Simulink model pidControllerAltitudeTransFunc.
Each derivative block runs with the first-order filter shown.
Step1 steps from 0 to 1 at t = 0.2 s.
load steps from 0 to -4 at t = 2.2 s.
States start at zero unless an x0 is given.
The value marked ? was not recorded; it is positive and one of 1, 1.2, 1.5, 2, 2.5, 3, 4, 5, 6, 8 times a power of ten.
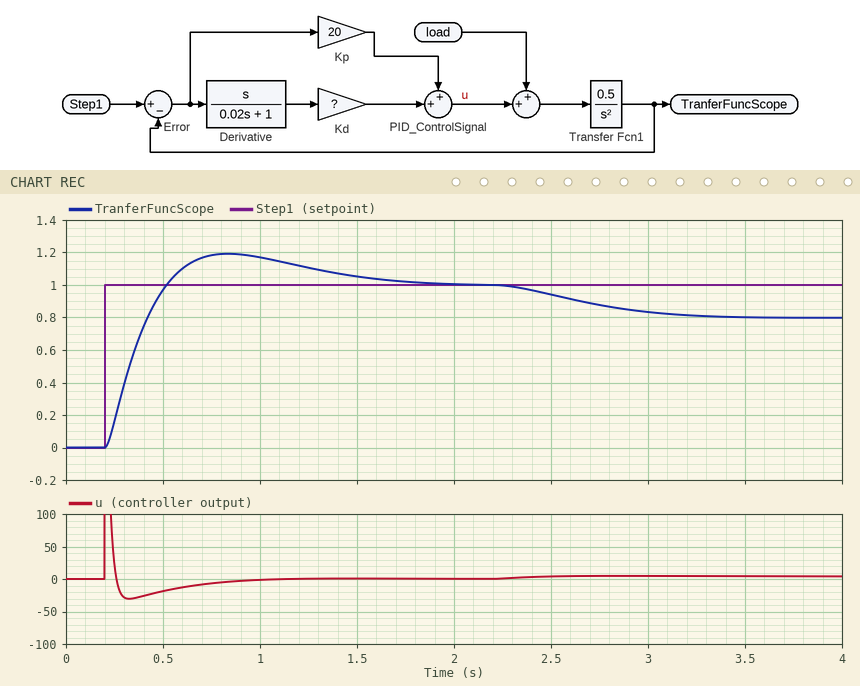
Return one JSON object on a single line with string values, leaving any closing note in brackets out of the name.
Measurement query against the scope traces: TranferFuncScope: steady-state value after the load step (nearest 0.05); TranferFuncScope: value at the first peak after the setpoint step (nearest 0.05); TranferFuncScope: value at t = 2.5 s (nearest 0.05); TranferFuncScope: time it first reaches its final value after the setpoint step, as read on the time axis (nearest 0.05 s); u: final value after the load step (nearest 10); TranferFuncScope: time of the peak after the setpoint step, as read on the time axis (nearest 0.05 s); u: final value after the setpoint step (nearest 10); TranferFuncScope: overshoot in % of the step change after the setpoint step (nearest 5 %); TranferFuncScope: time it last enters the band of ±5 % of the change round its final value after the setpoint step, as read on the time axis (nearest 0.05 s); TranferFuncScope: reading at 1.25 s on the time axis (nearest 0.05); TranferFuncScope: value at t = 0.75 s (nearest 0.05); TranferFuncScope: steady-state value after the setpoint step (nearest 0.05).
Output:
{"TranferFuncScope: steady-state value after the load step": "0.80", "TranferFuncScope: value at the first peak after the setpoint step": "1.20", "TranferFuncScope: value at t = 2.5 s": "0.95", "TranferFuncScope: time it first reaches its final value after the setpoint step, as read on the time axis": "0.50 s", "u: final value after the load step": "0", "TranferFuncScope: time of the peak after the setpoint step, as read on the time axis": "0.85 s", "u: final value after the setpoint step": "0", "TranferFuncScope: overshoot in % of the step change after the setpoint step": "20 %", "TranferFuncScope: time it last enters the band of ±5 % of the change round its final value after the setpoint step, as read on the time axis": "1.50 s", "TranferFuncScope: reading at 1.25 s on the time axis": "1.10", "TranferFuncScope: value at t = 0.75 s": "1.20", "TranferFuncScope: steady-state value after the setpoint step": "1.00"}
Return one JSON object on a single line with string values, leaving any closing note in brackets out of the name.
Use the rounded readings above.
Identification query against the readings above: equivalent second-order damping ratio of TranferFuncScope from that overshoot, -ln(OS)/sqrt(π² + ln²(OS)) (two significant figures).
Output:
{"equivalent second-order damping ratio of TranferFuncScope from that overshoot, -ln(OS)/sqrt(π² + ln²(OS))": "0.46"}
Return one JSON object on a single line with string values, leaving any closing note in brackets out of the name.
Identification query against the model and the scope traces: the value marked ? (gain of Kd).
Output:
{"the value marked ?": "10"}
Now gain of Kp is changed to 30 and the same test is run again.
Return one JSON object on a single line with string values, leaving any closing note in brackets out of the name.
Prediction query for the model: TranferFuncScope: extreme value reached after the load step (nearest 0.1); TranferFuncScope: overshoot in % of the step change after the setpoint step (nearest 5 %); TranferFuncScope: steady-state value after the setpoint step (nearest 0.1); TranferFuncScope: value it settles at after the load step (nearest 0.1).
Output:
{"TranferFuncScope: extreme value reached after the load step": "0.9", "TranferFuncScope: overshoot in % of the step change after the setpoint step": "25 %", "TranferFuncScope: steady-state value after the setpoint step": "1.0", "TranferFuncScope: value it settles at after the load step": "0.9"}
